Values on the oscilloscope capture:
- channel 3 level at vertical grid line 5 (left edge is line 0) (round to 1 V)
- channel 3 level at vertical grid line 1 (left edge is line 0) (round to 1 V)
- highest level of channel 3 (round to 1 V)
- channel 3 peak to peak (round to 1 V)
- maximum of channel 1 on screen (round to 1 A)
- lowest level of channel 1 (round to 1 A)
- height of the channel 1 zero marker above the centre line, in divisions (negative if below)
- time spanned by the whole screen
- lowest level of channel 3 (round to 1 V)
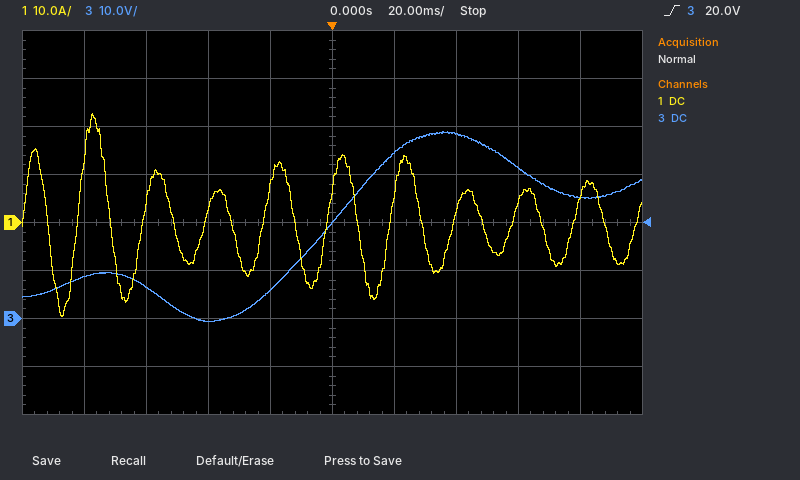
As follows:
20 V
9 V
39 V
40 V
23 A
-20 A
0.0 div
200 ms
-1 V
